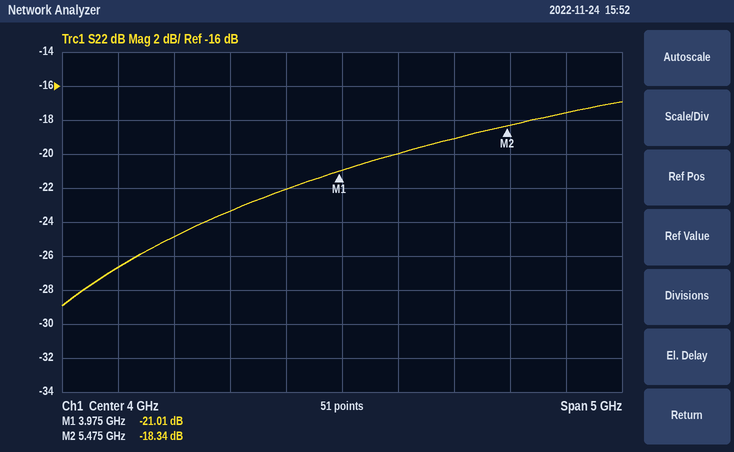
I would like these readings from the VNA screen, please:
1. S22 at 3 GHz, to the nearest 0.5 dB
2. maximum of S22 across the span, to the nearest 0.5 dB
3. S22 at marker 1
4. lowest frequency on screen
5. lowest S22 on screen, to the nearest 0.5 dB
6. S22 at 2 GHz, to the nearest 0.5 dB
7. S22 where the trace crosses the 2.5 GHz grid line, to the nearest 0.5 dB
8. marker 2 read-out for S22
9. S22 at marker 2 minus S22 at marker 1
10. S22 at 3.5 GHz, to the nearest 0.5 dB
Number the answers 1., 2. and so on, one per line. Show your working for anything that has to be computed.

1. -23.5 dB
2. -17.0 dB
3. -21.01 dB
4. 1.5 GHz
5. -29.0 dB
6. -26.5 dB
7. -25.0 dB
8. -18.34 dB
9. -18.34 − (-21.01) = 2.67 dB
10. -22.0 dB
